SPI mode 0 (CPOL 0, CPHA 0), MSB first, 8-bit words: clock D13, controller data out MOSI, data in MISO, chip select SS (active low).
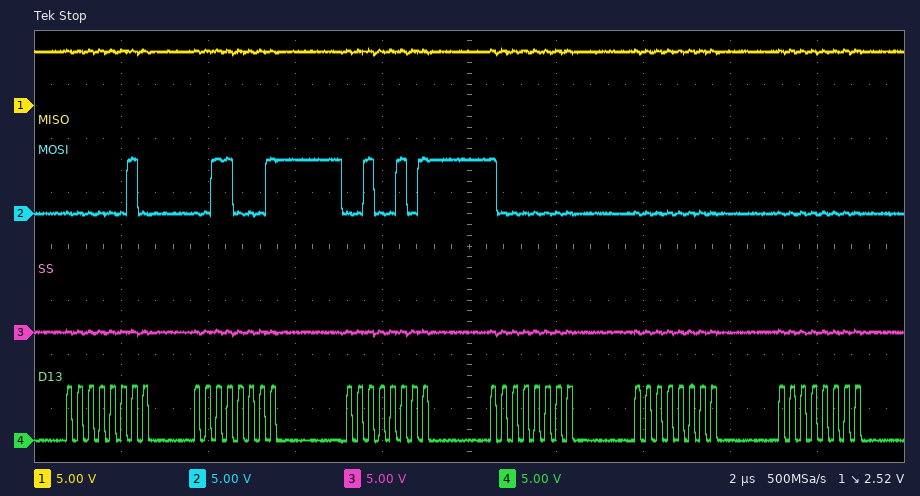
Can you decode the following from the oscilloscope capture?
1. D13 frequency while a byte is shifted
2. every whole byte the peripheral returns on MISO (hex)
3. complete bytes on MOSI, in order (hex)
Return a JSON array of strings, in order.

["4 MHz", "0xFF 0xFF 0xFF 0xFF 0xFF 0xFF", "0x02 0x31 0x25 0x80 0x00 0x00"]
